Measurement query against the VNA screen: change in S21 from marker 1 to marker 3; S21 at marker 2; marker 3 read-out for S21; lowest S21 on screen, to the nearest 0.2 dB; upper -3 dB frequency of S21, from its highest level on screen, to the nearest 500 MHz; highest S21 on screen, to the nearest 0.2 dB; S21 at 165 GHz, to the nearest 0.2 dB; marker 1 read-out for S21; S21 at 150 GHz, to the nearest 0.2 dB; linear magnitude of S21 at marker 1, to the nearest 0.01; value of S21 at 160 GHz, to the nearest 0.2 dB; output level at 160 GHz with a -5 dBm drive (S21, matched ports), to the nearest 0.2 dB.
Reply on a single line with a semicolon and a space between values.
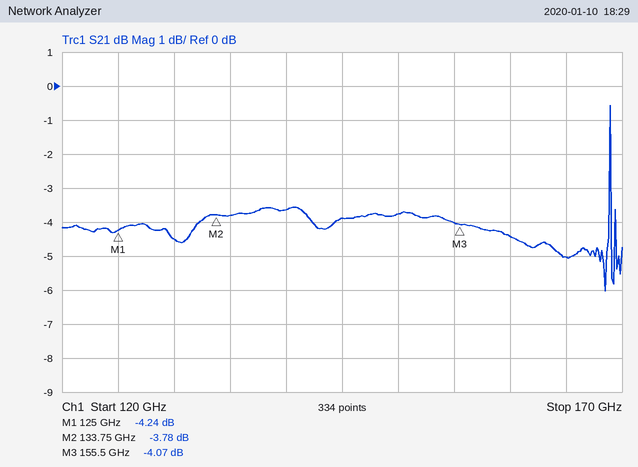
0.17 dB; -3.78 dB; -4.07 dB; -6.0 dB; 169.0 GHz; -0.6 dB; -5.0 dB; -4.24 dB; -3.8 dB; 0.61; -4.4 dB; -9.4 dBm
